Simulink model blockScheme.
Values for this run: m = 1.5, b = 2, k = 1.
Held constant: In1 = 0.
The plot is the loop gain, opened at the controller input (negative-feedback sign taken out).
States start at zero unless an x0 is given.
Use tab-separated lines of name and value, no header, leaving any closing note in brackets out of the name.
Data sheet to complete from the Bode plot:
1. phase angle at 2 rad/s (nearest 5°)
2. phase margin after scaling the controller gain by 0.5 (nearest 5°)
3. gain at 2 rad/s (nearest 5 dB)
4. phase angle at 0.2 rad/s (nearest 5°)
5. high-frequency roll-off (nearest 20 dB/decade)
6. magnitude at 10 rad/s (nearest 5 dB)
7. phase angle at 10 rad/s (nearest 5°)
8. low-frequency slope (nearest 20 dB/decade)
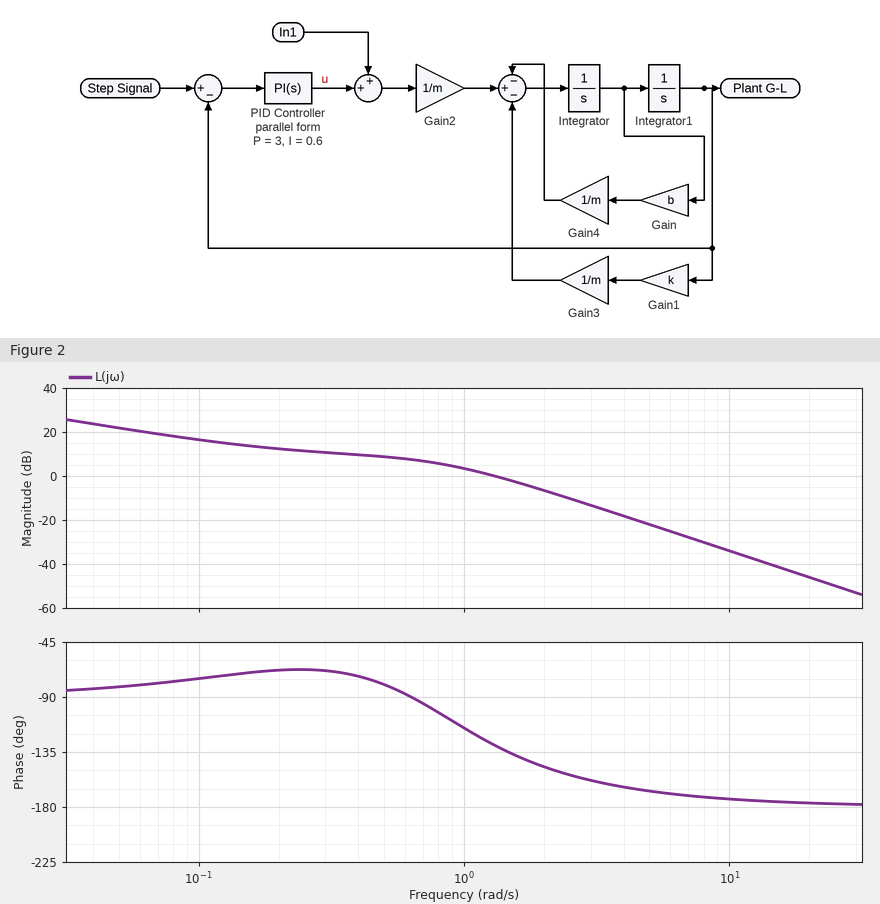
phase angle at 2 rad/s	-145°
phase margin after scaling the controller gain by 0.5	80°
gain at 2 rad/s	-5 dB
phase angle at 0.2 rad/s	-70°
high-frequency roll-off	-40 dB/decade
magnitude at 10 rad/s	-35 dB
phase angle at 10 rad/s	-175°
low-frequency slope	-20 dB/decade
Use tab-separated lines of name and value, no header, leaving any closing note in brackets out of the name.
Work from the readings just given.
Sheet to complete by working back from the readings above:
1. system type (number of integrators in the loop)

system type	1
